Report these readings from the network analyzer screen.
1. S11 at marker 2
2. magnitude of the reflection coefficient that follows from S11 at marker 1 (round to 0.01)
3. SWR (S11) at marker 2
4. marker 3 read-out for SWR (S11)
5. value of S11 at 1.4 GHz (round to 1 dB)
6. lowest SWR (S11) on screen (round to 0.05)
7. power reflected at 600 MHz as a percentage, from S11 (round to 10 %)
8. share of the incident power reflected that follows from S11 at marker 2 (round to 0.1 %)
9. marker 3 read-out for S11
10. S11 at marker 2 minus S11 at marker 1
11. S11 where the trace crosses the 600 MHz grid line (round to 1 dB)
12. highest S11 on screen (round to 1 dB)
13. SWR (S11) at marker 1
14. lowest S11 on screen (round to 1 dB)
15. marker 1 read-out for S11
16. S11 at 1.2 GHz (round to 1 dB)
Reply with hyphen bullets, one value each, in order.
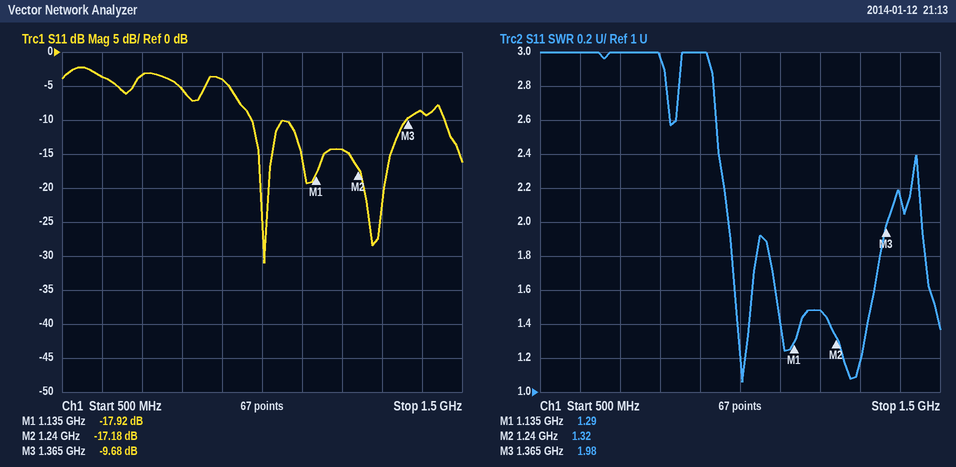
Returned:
- -17.18 dB
- 0.13
- 1.32
- 1.98
- -9 dB
- 1.05
- 40 %
- 1.9 %
- -9.68 dB
- 0.74 dB
- -4 dB
- -2 dB
- 1.29
- -31 dB
- -17.92 dB
- -14 dB
